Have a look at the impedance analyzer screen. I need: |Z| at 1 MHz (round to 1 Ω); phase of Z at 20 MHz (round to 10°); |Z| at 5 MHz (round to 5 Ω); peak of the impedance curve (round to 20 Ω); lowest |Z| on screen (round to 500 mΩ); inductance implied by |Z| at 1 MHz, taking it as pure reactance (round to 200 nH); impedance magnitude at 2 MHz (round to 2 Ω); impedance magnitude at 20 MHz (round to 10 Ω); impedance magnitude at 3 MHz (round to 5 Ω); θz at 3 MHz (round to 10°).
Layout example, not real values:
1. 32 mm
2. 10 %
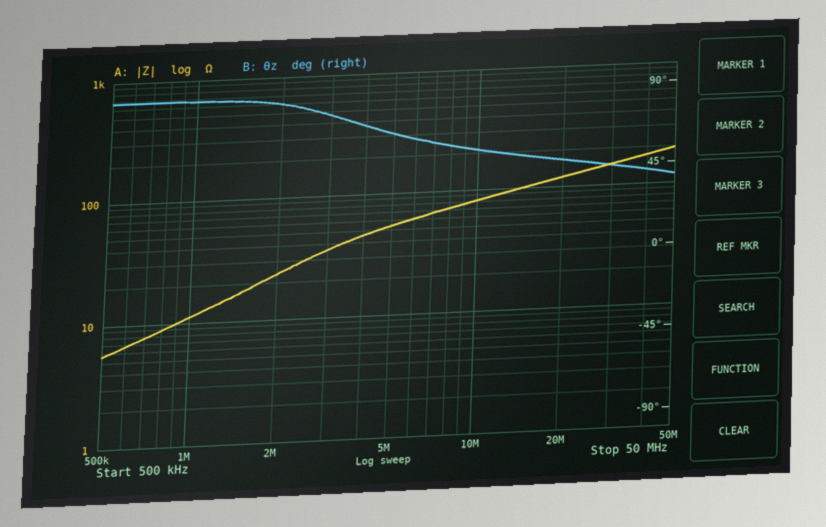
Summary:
1. 11 Ω
2. 50°
3. 55 Ω
4. 200 Ω
5. 5.5 Ω
6. 1.8 µH
7. 24 Ω
8. 120 Ω
9. 35 Ω
10. 80°
